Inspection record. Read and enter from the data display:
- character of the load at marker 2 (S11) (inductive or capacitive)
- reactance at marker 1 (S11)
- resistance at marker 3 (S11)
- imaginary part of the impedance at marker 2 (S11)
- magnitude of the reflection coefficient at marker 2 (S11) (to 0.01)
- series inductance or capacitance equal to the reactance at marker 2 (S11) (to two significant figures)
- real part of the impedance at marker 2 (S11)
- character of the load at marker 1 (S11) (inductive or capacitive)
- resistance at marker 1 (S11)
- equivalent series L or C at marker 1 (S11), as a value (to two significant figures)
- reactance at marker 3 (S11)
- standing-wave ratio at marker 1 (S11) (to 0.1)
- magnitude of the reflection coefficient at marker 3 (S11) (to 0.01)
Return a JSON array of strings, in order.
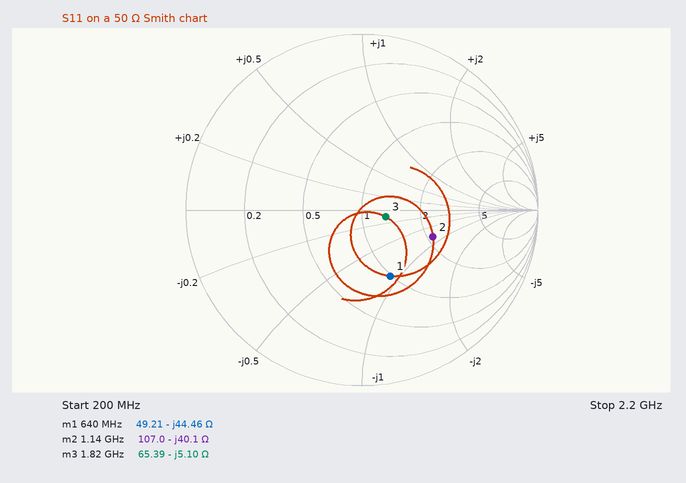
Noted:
["capacitive", "-44.46 Ω", "65.39 Ω", "-40.1 Ω", "0.43", "3.5 pF", "107.0 Ω", "capacitive", "49.21 Ω", "5.6 pF", "-5.10 Ω", "2.4", "0.14"]
